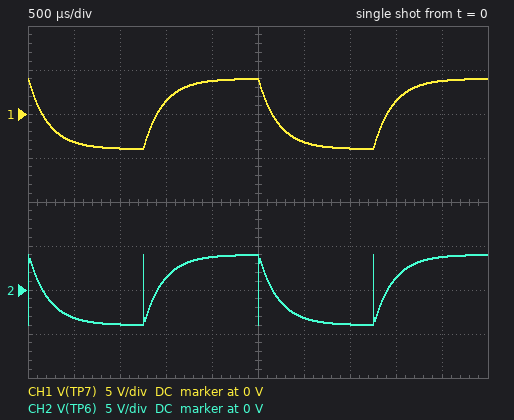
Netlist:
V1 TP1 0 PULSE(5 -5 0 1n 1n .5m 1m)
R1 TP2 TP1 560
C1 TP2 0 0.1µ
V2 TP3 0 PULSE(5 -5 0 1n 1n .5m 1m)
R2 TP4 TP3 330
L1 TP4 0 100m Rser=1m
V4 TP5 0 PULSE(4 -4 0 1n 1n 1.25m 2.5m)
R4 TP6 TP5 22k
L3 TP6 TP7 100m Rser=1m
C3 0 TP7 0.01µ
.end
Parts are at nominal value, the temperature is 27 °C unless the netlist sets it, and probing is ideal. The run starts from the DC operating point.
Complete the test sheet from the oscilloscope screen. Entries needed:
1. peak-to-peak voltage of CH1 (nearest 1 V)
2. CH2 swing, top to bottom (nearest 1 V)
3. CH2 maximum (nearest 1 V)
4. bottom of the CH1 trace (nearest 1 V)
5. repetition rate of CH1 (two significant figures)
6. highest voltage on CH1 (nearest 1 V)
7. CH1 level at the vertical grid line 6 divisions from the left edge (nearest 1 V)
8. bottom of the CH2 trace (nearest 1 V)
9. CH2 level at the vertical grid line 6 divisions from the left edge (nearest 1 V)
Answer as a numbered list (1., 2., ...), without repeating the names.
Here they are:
1. 8 V
2. 8 V
3. 4 V
4. -4 V
5. 400 Hz
6. 4 V
7. -3 V
8. -4 V
9. -3 V
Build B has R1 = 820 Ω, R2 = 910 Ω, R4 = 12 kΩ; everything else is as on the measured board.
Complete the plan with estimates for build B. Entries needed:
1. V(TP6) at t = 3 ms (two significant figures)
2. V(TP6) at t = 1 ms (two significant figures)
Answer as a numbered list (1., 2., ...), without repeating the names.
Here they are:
1. -3.9 V
2. -4.0 V
